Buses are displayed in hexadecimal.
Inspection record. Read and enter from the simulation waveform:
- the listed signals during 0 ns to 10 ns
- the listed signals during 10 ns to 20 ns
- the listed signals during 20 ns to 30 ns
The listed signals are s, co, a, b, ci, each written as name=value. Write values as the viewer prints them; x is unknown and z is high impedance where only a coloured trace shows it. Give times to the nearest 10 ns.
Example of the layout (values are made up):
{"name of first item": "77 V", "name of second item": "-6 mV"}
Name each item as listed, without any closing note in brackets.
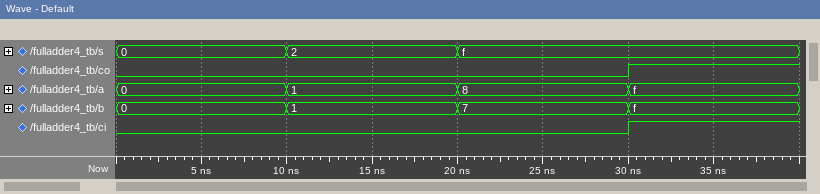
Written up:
{"the listed signals during 0 ns to 10 ns": "s=0, co=0, a=0, b=0, ci=0", "the listed signals during 10 ns to 20 ns": "s=2, co=0, a=1, b=1, ci=0", "the listed signals during 20 ns to 30 ns": "s=f, co=0, a=8, b=7, ci=0"}
